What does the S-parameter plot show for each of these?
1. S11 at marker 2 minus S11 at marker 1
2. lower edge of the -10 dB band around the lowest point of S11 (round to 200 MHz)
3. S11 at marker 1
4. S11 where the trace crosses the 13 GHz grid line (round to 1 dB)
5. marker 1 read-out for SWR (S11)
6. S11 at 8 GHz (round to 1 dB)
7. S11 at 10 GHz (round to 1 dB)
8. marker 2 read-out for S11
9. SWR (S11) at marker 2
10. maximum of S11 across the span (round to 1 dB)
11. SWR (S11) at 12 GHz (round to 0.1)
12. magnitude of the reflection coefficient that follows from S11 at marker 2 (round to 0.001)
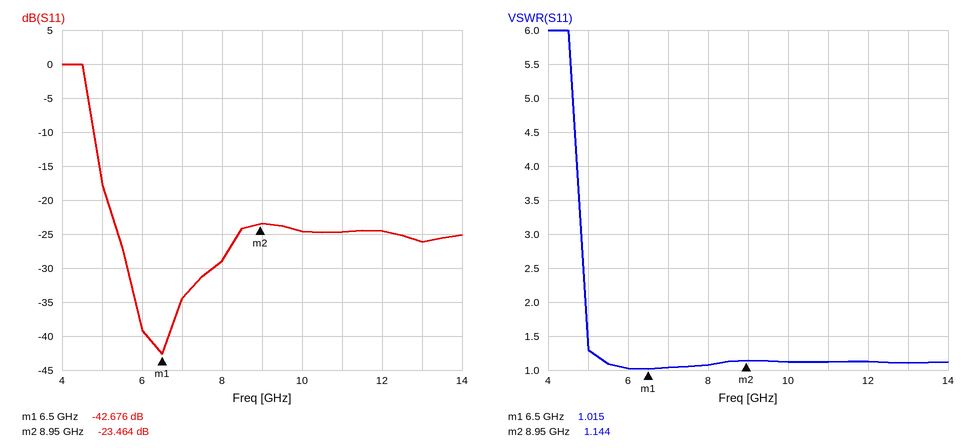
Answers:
19.212 dB
4.8 GHz
-42.676 dB
-26 dB
1.015
-29 dB
-25 dB
-23.464 dB
1.144
0 dB
1.1
0.067
